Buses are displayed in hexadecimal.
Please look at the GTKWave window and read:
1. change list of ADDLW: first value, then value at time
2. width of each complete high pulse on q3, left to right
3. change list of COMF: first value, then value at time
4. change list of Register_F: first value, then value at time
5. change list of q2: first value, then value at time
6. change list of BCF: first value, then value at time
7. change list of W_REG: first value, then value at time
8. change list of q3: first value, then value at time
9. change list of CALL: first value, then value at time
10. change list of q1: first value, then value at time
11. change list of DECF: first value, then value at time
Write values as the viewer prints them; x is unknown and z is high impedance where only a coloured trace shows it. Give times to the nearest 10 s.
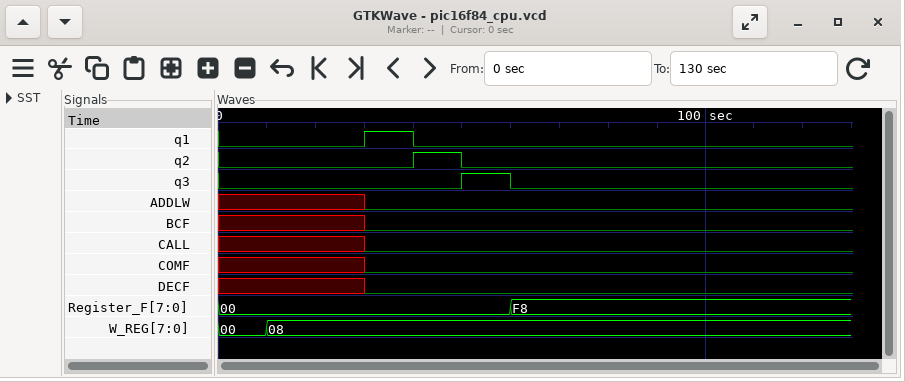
x, 0 at 30 s
10 s
x, 0 at 30 s
00, F8 at 60 s
0, 1 at 40 s, 0 at 50 s
x, 0 at 30 s
00, 08 at 10 s
0, 1 at 50 s, 0 at 60 s
x, 0 at 30 s
0, 1 at 30 s, 0 at 40 s
x, 0 at 30 s
